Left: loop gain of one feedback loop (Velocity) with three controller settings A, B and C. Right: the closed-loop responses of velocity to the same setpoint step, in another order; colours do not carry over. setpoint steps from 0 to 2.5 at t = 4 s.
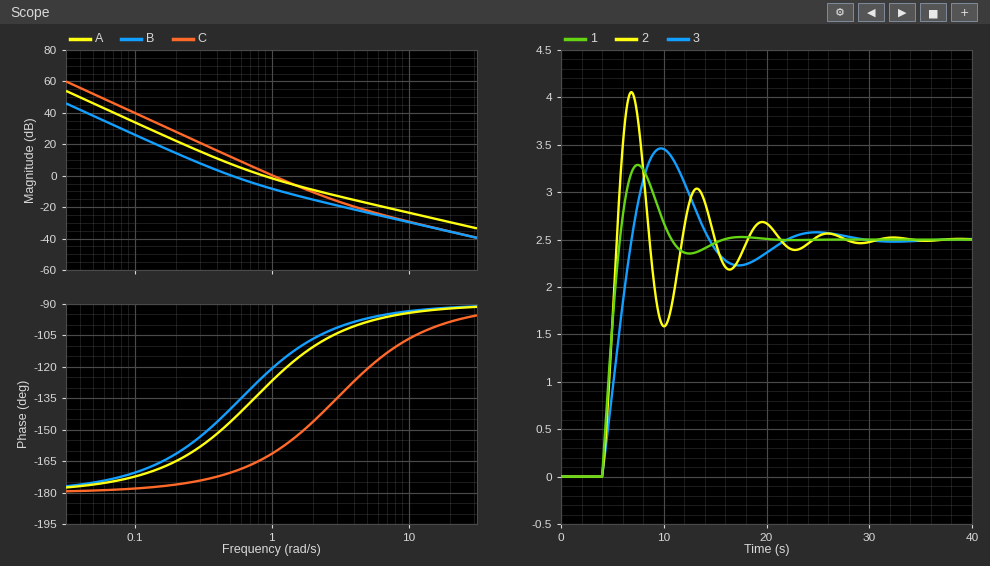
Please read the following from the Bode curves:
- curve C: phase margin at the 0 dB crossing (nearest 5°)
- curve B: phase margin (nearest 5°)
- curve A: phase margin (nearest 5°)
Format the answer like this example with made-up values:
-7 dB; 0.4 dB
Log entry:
20°; 40°; 50°
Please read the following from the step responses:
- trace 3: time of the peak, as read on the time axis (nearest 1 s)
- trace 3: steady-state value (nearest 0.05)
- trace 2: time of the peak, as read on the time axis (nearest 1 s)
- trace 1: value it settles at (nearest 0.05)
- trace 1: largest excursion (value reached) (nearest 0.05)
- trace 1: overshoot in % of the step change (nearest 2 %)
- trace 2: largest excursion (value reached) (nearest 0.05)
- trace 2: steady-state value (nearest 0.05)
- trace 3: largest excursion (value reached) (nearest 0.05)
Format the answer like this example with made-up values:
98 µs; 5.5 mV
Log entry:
10 s; 2.50; 7 s; 2.50; 3.30; 32 %; 4.05; 2.50; 3.45
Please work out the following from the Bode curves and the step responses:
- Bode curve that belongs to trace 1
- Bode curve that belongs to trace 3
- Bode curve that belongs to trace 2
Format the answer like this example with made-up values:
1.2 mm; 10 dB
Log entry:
A; B; C
